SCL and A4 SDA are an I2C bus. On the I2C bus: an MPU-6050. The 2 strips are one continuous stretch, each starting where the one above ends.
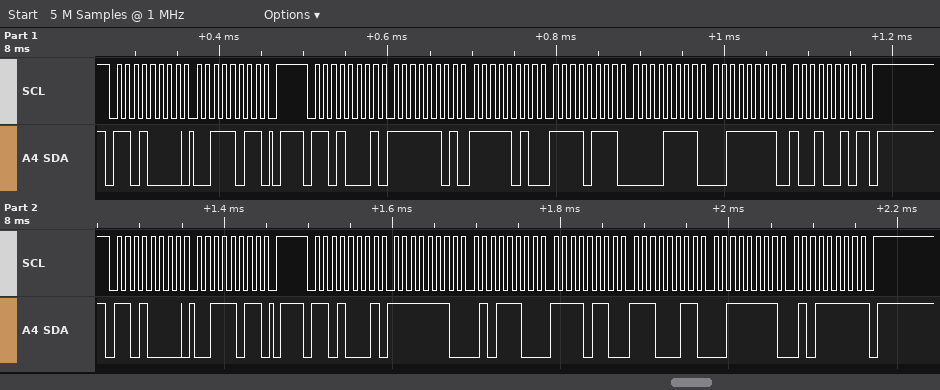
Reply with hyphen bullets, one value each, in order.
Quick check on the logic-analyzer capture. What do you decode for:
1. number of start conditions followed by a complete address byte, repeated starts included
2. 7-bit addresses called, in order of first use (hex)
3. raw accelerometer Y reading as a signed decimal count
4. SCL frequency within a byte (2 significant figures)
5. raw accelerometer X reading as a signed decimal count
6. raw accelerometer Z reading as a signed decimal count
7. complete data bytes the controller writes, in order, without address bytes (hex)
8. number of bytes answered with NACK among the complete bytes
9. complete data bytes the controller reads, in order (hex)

- 4
- 0x68
- -2289
- 100 kHz
- -518
- 16274
- 3B 3B
- 2
- FD FA F7 0F 3F 92 FE 5C F6 E3 3F 5F
